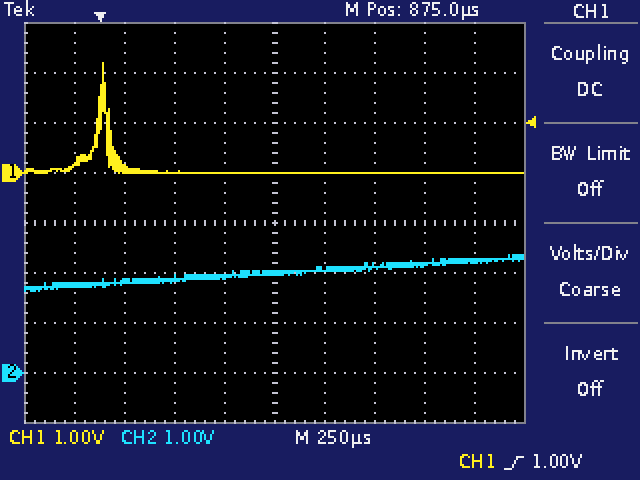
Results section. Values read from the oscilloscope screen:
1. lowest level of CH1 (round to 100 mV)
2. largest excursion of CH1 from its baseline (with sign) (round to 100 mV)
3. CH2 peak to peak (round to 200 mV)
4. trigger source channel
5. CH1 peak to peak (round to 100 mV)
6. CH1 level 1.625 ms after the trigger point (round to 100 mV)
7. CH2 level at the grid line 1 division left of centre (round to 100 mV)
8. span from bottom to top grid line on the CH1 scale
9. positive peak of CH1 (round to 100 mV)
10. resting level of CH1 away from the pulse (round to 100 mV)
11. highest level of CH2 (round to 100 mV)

0.0 V
+2.2 V
800 mV
CH1
2.2 V
0.0 V
1.9 V
8 V
2.2 V
0.0 V
2.4 V
